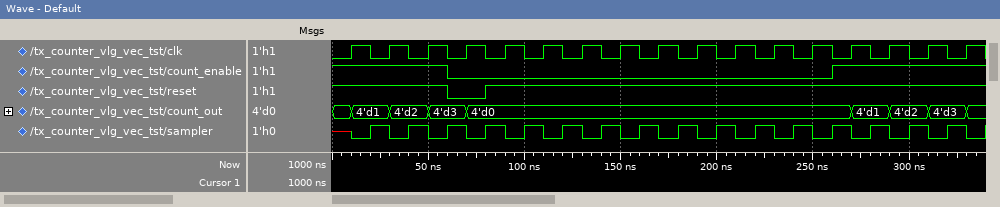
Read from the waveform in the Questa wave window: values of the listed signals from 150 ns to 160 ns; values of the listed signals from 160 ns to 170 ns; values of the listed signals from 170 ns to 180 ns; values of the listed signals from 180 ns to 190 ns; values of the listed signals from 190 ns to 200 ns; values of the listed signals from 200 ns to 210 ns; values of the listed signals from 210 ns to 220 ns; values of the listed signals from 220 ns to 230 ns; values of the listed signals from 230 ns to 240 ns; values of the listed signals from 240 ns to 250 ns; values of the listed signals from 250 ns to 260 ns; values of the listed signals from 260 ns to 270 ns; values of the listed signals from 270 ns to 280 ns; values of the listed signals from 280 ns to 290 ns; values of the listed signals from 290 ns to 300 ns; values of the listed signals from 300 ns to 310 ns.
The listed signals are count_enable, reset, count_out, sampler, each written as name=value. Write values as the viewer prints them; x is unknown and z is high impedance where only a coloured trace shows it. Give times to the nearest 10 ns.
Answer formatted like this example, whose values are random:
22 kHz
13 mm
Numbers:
count_enable=0, reset=1, count_out=4'd0, sampler=0
count_enable=0, reset=1, count_out=4'd0, sampler=1
count_enable=0, reset=1, count_out=4'd0, sampler=0
count_enable=0, reset=1, count_out=4'd0, sampler=1
count_enable=0, reset=1, count_out=4'd0, sampler=0
count_enable=0, reset=1, count_out=4'd0, sampler=1
count_enable=0, reset=1, count_out=4'd0, sampler=0
count_enable=0, reset=1, count_out=4'd0, sampler=1
count_enable=0, reset=1, count_out=4'd0, sampler=0
count_enable=0, reset=1, count_out=4'd0, sampler=1
count_enable=0, reset=1, count_out=4'd0, sampler=0
count_enable=1, reset=1, count_out=4'd0, sampler=1
count_enable=1, reset=1, count_out=4'd1, sampler=0
count_enable=1, reset=1, count_out=4'd1, sampler=1
count_enable=1, reset=1, count_out=4'd2, sampler=0
count_enable=1, reset=1, count_out=4'd2, sampler=1
